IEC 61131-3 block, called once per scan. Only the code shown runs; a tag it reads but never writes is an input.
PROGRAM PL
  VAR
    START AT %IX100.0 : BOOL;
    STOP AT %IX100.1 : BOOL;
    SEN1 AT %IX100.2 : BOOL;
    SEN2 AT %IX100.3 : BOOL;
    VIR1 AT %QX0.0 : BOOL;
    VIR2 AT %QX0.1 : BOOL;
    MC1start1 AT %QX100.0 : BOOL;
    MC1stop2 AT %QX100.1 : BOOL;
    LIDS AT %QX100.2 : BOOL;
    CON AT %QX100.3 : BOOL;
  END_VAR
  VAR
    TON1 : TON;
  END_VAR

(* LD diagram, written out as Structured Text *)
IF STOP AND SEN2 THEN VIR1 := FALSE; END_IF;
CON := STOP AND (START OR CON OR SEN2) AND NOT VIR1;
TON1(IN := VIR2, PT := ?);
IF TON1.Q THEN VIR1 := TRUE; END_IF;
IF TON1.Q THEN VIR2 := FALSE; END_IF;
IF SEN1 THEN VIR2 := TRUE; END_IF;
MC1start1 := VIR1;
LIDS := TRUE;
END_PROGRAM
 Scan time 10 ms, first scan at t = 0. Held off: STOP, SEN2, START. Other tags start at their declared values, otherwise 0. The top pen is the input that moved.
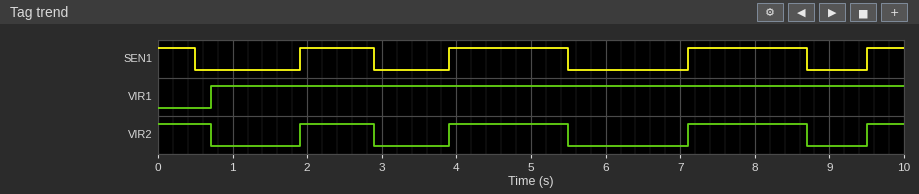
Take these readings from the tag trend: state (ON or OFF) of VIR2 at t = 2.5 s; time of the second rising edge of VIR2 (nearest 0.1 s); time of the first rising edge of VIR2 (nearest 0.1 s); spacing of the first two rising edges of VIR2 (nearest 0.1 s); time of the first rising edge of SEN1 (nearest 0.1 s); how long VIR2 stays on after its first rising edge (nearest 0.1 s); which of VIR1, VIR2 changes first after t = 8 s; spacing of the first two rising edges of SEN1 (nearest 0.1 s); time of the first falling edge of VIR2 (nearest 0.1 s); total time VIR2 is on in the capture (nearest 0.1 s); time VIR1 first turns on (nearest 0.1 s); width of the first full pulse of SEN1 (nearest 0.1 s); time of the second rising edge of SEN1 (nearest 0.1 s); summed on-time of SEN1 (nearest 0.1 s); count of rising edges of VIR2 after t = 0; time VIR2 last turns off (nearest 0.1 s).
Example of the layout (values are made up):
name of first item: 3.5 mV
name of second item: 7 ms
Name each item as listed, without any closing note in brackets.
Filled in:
state (ON or OFF) of VIR2 at t = 2.5 s: ON
time of the second rising edge of VIR2: 3.9 s
time of the first rising edge of VIR2: 1.9 s
spacing of the first two rising edges of VIR2: 2.0 s
time of the first rising edge of SEN1: 1.9 s
how long VIR2 stays on after its first rising edge: 1.0 s
which of VIR1, VIR2 changes first after t = 8 s: VIR2
spacing of the first two rising edges of SEN1: 2.0 s
time of the first falling edge of VIR2: 0.7 s
total time VIR2 is on in the capture: 5.4 s
time VIR1 first turns on: 0.7 s
width of the first full pulse of SEN1: 1.0 s
time of the second rising edge of SEN1: 3.9 s
summed on-time of SEN1: 5.2 s
count of rising edges of VIR2 after t = 0: 4
time VIR2 last turns off: 8.7 s
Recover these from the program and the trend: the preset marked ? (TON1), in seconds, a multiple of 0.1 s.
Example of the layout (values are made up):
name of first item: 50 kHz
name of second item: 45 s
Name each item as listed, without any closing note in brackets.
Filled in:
the preset marked ? (TON1), in seconds, a multiple of 0.1 s: 0.7 s
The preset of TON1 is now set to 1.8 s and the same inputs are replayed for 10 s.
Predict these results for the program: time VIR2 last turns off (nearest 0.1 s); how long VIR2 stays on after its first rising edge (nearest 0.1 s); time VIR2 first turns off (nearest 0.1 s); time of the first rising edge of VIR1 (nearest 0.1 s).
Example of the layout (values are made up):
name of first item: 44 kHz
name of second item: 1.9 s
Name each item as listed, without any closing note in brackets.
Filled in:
time VIR2 last turns off: 8.9 s
how long VIR2 stays on after its first rising edge: 1.8 s
time VIR2 first turns off: 1.8 s
time of the first rising edge of VIR1: 1.8 s
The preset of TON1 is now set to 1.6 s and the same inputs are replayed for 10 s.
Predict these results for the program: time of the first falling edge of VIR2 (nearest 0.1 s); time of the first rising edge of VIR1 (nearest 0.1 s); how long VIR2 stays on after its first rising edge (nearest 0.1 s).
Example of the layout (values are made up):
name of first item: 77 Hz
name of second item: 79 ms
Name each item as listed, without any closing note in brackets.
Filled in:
time of the first falling edge of VIR2: 1.6 s
time of the first rising edge of VIR1: 1.6 s
how long VIR2 stays on after its first rising edge: 1.6 s
